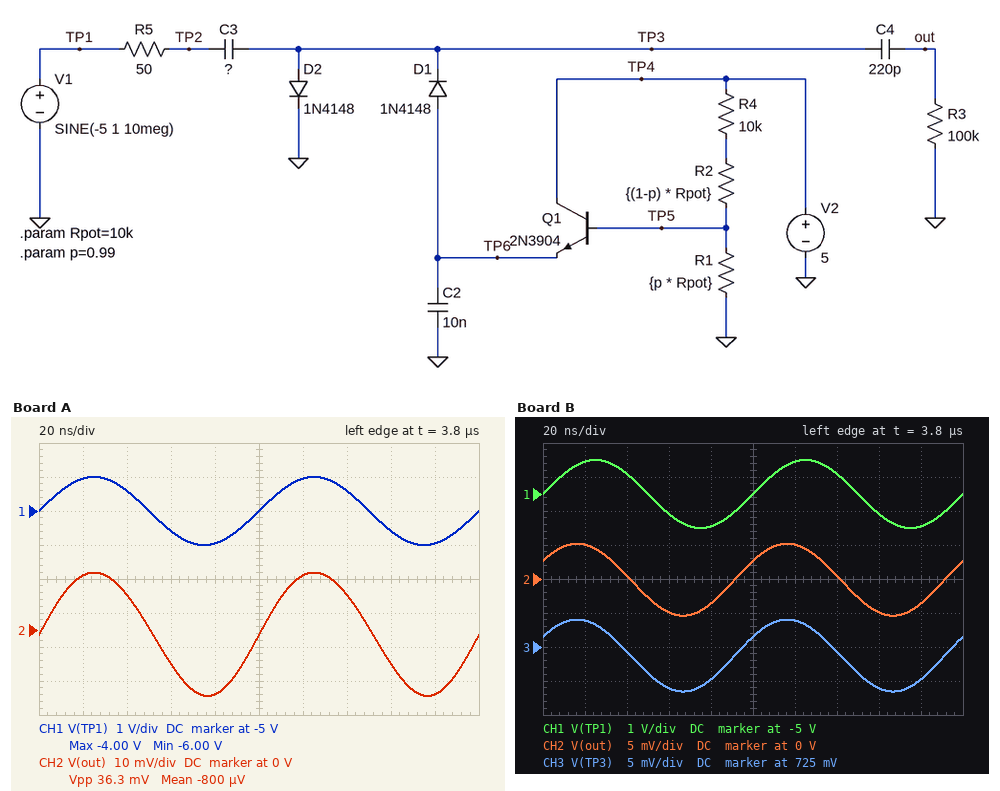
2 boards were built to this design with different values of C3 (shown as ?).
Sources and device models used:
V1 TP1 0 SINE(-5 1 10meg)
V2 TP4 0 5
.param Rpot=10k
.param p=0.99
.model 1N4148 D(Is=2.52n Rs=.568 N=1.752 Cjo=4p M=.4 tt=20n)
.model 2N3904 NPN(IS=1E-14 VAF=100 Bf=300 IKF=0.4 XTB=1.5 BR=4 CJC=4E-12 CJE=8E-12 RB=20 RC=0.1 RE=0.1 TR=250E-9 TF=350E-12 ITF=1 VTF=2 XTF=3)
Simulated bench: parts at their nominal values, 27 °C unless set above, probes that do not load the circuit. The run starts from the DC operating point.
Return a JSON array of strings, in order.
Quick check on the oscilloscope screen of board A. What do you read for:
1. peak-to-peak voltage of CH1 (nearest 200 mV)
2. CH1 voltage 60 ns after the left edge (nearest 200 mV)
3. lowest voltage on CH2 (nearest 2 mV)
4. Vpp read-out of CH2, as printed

["2.0 V", "-5.6 V", "-20 mV", "36.3 mV"]
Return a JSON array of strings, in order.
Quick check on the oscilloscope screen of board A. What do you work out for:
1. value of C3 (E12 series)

["330 pF"]
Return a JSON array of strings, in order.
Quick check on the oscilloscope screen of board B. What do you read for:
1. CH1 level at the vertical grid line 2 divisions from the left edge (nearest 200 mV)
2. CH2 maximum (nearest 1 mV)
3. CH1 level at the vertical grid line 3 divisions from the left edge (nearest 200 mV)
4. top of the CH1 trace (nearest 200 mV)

["-4.4 V", "5 mV", "-5.6 V", "-4.0 V"]
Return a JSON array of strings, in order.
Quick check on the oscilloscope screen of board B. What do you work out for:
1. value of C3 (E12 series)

["68 pF"]
